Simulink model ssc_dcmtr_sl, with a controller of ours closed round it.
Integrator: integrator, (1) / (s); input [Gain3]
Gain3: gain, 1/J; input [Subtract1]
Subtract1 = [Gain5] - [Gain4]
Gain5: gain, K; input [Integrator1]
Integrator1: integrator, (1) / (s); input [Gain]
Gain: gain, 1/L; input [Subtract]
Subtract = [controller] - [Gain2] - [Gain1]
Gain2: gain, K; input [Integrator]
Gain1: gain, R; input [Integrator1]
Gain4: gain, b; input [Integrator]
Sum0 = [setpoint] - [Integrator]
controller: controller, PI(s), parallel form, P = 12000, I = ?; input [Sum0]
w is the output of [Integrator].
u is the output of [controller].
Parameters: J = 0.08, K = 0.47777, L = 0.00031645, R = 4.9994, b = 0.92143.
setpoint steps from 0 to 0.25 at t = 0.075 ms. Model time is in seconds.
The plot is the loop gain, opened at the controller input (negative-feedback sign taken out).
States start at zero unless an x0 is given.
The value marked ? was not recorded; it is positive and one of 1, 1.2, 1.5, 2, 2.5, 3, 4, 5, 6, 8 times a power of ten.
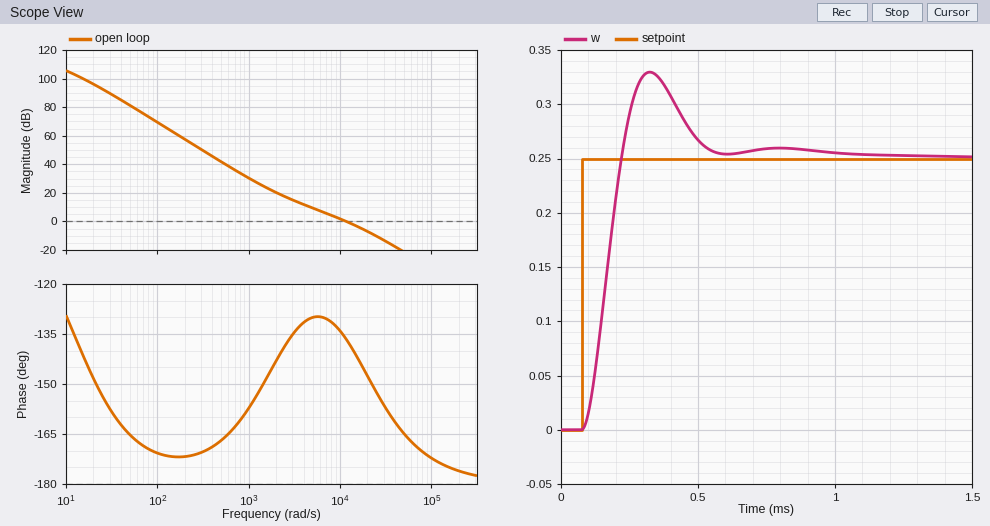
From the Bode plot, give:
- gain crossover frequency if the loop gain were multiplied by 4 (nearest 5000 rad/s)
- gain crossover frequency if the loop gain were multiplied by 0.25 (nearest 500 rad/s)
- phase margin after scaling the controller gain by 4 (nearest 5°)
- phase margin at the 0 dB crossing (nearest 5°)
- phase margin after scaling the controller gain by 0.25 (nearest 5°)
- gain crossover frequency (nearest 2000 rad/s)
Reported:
30000 rad/s
4000 rad/s
25°
45°
50°
12000 rad/s
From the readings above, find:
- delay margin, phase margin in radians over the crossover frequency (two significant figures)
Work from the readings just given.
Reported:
0.000065 s
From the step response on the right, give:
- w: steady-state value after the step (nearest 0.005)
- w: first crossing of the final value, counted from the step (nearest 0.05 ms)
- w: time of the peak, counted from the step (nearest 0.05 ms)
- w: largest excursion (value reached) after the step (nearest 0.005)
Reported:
0.250
0.15 ms
0.25 ms
0.330
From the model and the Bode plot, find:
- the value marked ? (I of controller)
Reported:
2.5e+07
